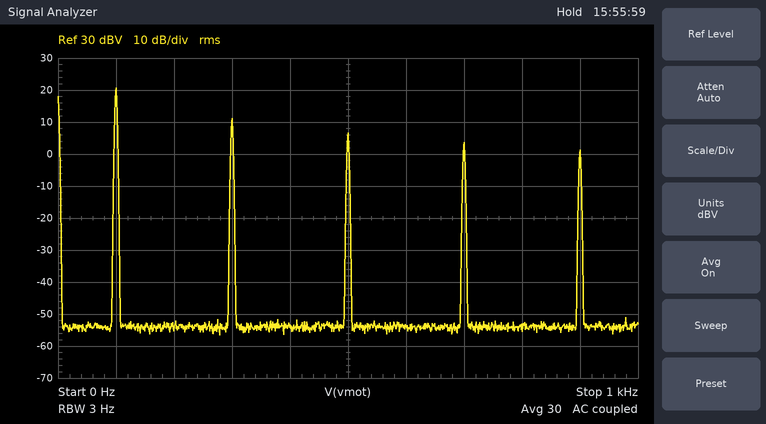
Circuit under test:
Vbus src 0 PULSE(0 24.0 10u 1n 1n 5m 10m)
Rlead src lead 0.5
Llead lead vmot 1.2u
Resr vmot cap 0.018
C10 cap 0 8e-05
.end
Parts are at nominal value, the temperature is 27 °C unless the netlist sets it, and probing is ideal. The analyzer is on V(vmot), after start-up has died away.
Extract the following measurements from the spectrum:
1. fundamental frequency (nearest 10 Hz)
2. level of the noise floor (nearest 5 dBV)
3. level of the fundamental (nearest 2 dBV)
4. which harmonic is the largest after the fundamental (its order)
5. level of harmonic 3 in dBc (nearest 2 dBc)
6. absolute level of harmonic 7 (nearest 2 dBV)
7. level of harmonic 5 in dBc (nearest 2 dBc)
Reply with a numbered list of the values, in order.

1. 100 Hz
2. -55 dBV
3. 20 dBV
4. 3
5. -10 dBc
6. 4 dBV
7. -14 dBc
